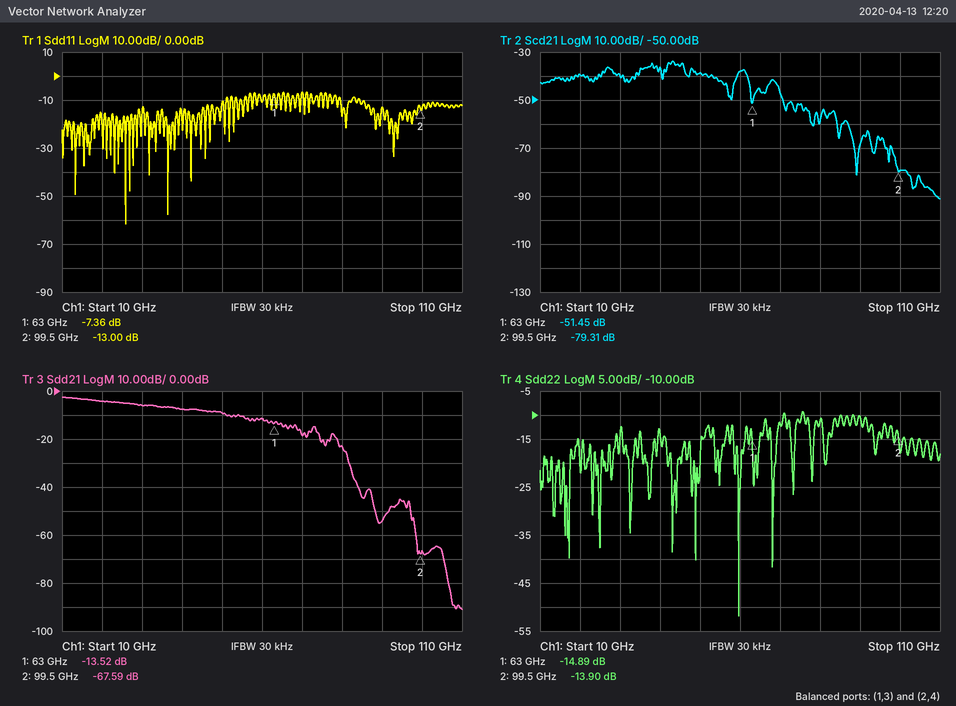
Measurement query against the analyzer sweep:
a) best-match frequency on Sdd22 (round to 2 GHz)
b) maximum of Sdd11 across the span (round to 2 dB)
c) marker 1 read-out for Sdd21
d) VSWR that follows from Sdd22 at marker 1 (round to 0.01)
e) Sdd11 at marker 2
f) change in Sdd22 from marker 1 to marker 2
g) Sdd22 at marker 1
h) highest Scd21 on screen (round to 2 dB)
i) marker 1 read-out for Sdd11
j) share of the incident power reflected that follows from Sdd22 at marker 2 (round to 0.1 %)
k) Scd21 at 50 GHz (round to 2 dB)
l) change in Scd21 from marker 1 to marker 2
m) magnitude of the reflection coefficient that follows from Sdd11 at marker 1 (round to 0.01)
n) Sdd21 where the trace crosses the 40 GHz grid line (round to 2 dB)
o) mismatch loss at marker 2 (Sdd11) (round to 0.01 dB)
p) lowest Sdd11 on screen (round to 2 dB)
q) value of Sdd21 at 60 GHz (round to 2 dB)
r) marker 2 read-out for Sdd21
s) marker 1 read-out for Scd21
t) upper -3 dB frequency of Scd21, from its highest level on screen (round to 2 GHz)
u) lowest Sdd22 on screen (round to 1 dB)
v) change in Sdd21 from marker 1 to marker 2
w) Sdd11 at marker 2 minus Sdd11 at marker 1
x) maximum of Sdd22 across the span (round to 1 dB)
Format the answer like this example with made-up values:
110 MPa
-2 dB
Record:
60 GHz
-6 dB
-13.52 dB
1.44
-13.00 dB
0.99 dB
-14.89 dB
-34 dB
-7.36 dB
4.1 %
-38 dB
-27.86 dB
0.43
-8 dB
0.22 dB
-62 dB
-12 dB
-67.59 dB
-51.45 dB
46 GHz
-52 dB
-54.07 dB
-5.64 dB
-9 dB
